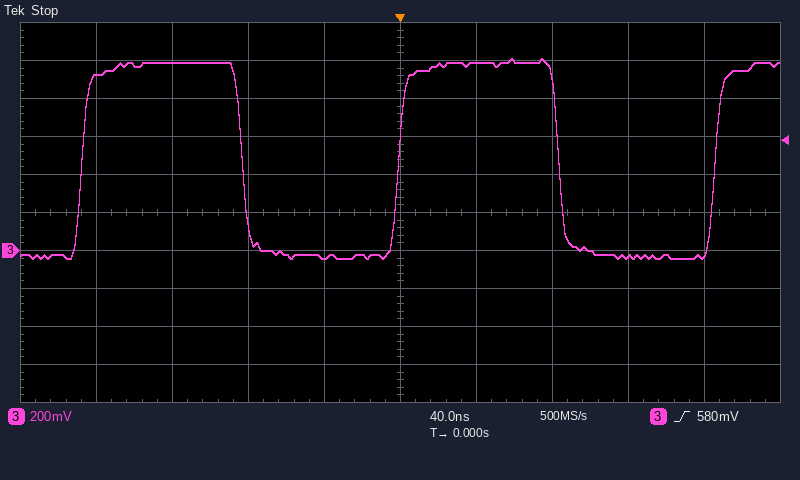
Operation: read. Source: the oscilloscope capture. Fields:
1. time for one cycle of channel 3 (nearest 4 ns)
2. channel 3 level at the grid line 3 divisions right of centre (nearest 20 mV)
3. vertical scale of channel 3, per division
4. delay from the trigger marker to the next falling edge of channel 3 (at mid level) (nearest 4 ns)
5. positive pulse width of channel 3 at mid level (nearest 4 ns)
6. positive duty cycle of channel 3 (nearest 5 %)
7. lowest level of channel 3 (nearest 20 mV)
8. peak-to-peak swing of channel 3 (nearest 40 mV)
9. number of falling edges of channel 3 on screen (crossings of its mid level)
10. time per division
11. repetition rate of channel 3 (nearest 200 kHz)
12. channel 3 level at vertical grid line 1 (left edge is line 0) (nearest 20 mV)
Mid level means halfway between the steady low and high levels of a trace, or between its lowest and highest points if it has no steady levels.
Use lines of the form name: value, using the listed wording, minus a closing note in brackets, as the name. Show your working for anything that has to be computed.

time for one cycle of channel 3: 168 ns
channel 3 level at the grid line 3 divisions right of centre: -40 mV
vertical scale of channel 3, per division: 200 mV
delay from the trigger marker to the next falling edge of channel 3 (at mid level): 84 ns
positive pulse width of channel 3 at mid level: 84 ns
positive duty cycle of channel 3: 84 ns / 168 ns ≈ 50 %
lowest level of channel 3: -40 mV
peak-to-peak swing of channel 3: 1.04 V
number of falling edges of channel 3 on screen: 2
time per division: 40 ns
repetition rate of channel 3: 1 / 168 ns ≈ 6.0 MHz
channel 3 level at vertical grid line 1 (left edge is line 0): 920 mV
